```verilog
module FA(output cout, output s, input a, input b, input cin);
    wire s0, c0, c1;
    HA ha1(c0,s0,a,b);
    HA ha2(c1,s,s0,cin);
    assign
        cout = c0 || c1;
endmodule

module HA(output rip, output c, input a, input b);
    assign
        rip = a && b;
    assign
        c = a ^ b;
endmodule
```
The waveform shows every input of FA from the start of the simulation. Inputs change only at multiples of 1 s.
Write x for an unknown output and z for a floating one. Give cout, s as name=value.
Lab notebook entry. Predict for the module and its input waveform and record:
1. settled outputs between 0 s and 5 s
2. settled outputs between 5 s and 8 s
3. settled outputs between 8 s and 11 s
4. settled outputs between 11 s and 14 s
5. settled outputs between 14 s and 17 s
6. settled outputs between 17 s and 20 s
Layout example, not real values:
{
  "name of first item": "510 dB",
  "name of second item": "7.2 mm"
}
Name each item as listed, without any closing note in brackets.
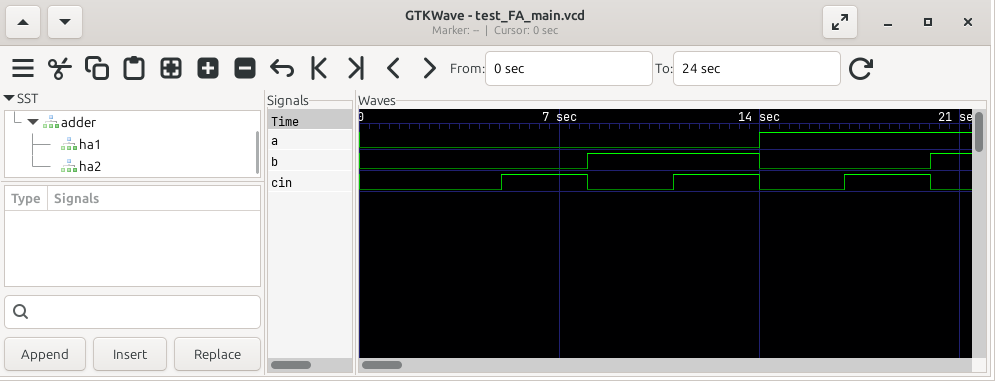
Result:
{
  "settled outputs between 0 s and 5 s": "cout=0, s=0",
  "settled outputs between 5 s and 8 s": "cout=0, s=1",
  "settled outputs between 8 s and 11 s": "cout=0, s=1",
  "settled outputs between 11 s and 14 s": "cout=1, s=0",
  "settled outputs between 14 s and 17 s": "cout=0, s=1",
  "settled outputs between 17 s and 20 s": "cout=1, s=0"
}
